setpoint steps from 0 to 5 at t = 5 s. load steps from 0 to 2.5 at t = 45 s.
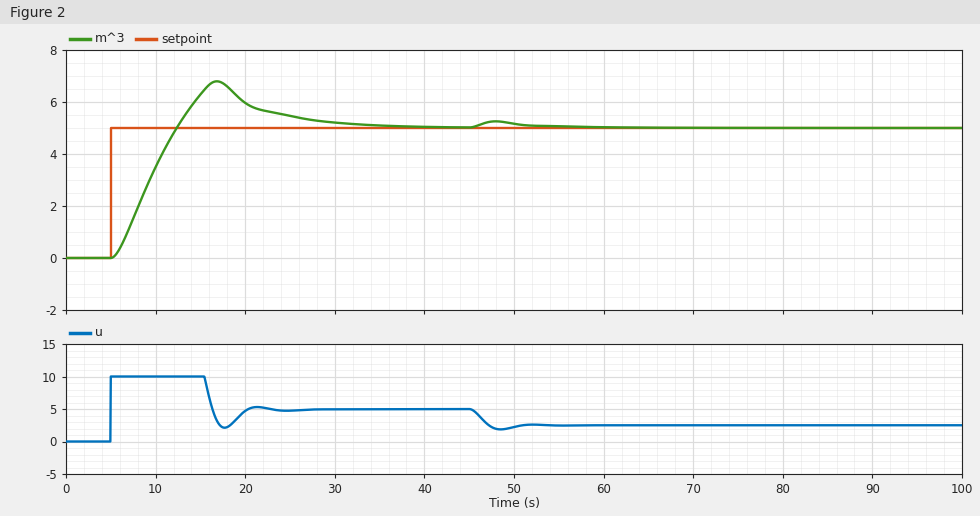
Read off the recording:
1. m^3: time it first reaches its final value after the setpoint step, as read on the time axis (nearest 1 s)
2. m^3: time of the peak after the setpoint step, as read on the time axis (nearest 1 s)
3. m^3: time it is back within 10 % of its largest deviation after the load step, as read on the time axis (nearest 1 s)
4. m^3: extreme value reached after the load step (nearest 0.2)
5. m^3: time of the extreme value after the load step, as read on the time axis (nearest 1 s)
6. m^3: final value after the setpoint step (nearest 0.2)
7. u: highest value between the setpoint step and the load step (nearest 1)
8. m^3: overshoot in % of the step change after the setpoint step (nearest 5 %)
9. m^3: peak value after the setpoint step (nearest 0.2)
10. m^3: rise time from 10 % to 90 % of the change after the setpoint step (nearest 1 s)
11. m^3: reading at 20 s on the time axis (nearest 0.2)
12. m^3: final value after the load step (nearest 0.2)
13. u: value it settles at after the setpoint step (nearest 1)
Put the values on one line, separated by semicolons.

12 s; 17 s; 62 s; 5.2; 48 s; 5.0; 10; 35 %; 6.8; 5 s; 6.0; 5.0; 5
